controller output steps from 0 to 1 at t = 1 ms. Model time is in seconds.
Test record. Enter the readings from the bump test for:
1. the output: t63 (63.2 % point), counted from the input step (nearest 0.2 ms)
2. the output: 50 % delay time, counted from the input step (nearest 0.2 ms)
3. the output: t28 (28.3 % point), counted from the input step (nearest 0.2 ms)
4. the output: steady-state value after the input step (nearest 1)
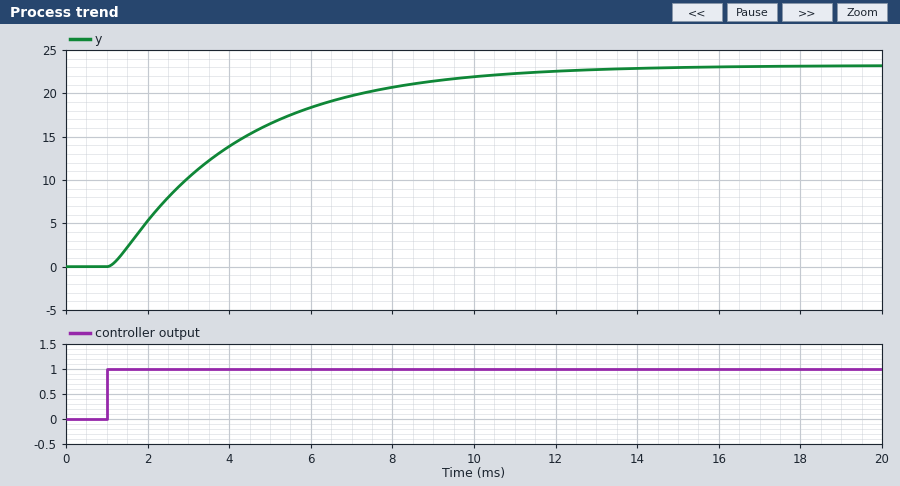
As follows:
3.2 ms
2.4 ms
1.2 ms
23
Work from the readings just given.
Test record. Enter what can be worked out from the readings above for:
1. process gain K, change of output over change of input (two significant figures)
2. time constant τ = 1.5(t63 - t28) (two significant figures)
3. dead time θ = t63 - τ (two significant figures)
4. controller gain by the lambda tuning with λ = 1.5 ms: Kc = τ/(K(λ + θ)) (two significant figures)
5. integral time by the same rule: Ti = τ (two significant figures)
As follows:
23
3.0 ms
0.20 ms
0.077
3.0 ms
